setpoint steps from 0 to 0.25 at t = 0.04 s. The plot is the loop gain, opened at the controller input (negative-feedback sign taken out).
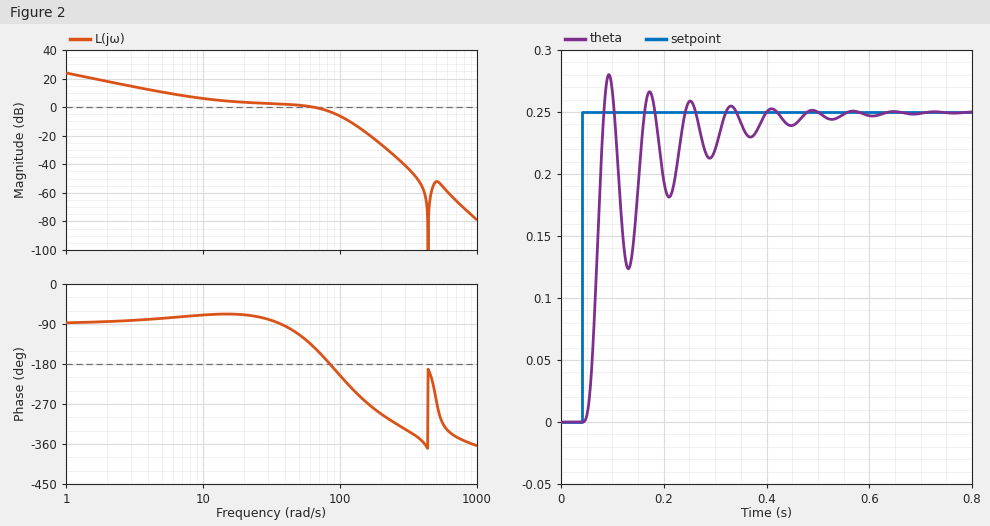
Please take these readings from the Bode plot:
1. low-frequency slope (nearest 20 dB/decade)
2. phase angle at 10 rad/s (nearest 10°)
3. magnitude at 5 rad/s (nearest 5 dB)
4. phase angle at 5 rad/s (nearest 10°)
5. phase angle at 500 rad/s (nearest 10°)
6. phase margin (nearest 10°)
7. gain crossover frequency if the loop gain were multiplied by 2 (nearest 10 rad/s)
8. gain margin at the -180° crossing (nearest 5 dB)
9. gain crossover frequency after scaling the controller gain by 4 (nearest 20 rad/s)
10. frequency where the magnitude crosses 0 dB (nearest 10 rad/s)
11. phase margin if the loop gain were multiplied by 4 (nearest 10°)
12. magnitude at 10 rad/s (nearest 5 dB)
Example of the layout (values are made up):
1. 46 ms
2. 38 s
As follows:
1. -20 dB/decade
2. -70°
3. 10 dB
4. -80°
5. -260°
6. 40°
7. 100 rad/s
8. 5 dB
9. 120 rad/s
10. 60 rad/s
11. -60°
12. 5 dB
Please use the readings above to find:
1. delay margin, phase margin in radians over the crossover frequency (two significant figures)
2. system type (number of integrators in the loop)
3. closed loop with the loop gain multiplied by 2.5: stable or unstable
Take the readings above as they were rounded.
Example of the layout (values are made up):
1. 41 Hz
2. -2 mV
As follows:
1. 0.012 s
2. 1
3. unstable
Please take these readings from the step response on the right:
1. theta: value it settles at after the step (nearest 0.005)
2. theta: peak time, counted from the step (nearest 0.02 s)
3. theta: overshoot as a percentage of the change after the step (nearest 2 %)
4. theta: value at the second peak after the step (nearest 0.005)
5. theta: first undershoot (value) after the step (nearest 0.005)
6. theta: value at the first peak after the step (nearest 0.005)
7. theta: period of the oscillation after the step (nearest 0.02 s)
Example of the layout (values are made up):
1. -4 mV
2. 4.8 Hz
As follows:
1. 0.250
2. 0.06 s
3. 12 %
4. 0.265
5. 0.125
6. 0.280
7. 0.08 s
